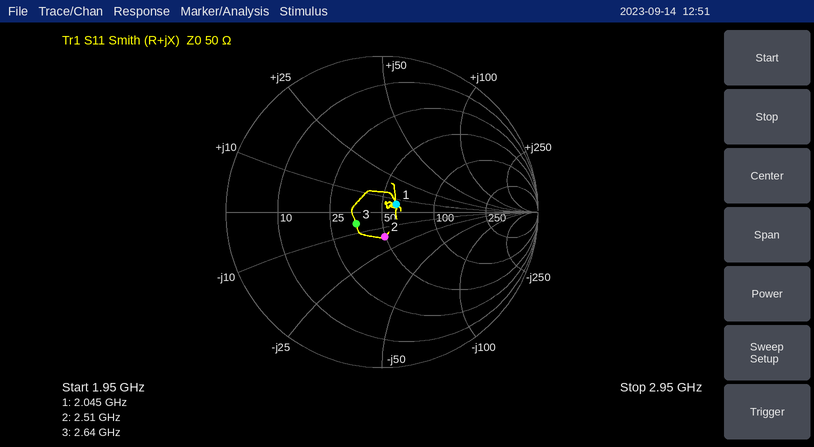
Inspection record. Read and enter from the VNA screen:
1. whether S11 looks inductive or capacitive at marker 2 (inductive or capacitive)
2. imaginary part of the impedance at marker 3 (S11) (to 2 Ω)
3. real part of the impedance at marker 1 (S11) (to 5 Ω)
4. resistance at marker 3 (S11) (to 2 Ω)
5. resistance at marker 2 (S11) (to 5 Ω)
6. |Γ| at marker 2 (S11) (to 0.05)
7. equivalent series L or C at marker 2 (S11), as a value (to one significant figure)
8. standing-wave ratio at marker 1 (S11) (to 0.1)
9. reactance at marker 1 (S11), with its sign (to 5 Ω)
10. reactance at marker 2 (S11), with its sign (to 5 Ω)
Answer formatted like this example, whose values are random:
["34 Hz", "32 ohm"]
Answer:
["capacitive", "-6 Ω", "60 Ω", "36 Ω", "50 Ω", "0.15", "4 pF", "1.2", "+5 Ω", "-15 Ω"]
